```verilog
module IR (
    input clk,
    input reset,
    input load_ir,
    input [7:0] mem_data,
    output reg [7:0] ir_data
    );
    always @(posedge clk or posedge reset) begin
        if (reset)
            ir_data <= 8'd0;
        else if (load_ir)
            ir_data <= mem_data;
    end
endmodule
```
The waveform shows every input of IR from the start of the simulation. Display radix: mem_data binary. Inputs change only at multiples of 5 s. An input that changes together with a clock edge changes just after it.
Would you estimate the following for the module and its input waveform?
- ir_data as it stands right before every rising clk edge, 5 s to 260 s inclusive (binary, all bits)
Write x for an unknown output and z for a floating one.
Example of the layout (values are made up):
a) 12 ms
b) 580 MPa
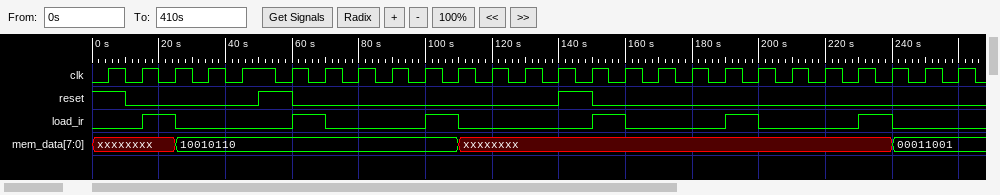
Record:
a) 00000000, 00000000, 00000000, x, x, 00000000, 00000000, 10010110, 10010110, 10010110, 10010110, 10010110, 10010110, 10010110, 00000000, 00000000, x, x, x, x, x, x, x, x, x, x
